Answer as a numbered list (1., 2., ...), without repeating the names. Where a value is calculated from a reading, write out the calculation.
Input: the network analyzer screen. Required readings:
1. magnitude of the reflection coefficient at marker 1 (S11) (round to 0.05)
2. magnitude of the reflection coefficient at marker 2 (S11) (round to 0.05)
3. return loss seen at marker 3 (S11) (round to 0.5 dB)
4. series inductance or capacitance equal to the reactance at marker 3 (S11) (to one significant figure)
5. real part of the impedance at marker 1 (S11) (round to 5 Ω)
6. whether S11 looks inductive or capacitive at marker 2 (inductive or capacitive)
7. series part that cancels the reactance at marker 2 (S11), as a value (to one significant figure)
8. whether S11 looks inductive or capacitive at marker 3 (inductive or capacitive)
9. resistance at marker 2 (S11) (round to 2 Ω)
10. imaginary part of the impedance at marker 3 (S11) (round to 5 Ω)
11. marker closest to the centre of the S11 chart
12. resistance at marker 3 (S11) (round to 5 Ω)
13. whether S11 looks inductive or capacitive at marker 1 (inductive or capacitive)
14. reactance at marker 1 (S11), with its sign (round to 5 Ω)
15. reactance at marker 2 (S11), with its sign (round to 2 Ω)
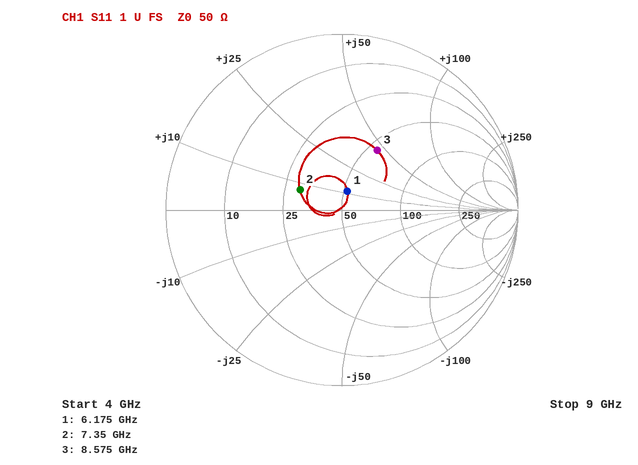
1. 0.10
2. 0.25
3. 8.0 dB
4. L = 45 Ω/(2π × 8.575 GHz) ≈ 835 pH, so 800 pH to one significant figure
5. 50 Ω
6. inductive
7. C = 1/(2π × 7.35 GHz × 8 Ω) ≈ 3 pF
8. inductive
9. 30 Ω
10. +45 Ω
11. marker 1
12. 55 Ω
13. inductive
14. +10 Ω
15. +8 Ω
